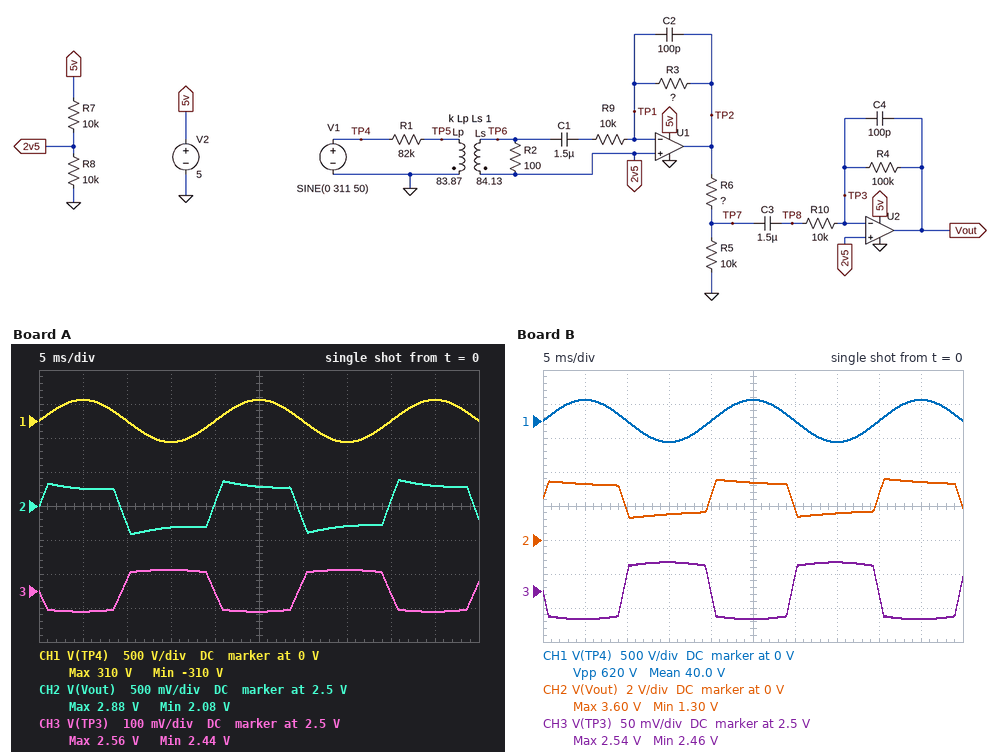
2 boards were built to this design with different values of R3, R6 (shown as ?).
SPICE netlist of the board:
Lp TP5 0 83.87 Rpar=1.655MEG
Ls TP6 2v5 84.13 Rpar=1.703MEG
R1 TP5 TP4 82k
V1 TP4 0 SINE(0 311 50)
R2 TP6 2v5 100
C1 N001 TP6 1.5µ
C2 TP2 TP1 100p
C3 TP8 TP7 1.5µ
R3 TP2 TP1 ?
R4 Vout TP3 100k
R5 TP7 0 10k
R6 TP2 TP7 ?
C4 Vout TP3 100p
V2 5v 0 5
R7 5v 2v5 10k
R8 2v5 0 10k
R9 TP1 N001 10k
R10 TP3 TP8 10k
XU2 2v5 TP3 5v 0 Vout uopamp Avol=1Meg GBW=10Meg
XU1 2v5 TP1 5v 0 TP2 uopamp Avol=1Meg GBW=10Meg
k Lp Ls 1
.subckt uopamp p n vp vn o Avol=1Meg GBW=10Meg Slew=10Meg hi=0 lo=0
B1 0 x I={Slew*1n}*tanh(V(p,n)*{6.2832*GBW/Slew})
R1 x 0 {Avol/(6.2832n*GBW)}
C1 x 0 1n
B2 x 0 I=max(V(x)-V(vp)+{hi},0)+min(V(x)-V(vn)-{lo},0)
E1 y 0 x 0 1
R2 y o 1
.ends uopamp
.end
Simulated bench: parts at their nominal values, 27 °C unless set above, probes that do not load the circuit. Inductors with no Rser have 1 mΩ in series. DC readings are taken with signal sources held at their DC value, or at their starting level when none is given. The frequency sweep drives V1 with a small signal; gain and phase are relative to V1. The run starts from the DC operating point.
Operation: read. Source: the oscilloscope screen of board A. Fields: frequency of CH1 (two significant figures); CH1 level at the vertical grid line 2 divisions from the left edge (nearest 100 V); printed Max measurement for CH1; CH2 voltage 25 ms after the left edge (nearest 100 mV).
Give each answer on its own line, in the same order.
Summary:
50 Hz
0 V
310 V
2.8 V
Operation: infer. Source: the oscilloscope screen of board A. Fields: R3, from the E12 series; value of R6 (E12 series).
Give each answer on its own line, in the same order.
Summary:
220 kΩ
180 kΩ
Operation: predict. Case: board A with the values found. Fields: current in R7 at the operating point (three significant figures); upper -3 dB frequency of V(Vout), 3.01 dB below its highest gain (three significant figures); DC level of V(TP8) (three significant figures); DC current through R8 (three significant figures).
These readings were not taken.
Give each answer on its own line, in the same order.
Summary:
250 µA
19.0 kHz
2.50 V
250 µA
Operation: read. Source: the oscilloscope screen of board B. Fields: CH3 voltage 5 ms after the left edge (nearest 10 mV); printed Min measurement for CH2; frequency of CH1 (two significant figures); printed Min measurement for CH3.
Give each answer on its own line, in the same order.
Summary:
2.46 V
1.30 V
50 Hz
2.46 V
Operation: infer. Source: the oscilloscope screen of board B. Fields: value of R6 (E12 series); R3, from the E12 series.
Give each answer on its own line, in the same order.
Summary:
100 kΩ
330 kΩ
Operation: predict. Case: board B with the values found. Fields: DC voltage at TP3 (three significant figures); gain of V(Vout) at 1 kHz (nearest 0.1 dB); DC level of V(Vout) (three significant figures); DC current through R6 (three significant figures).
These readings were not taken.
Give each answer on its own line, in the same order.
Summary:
2.50 V
-36.4 dB
2.50 V
22.7 µA
